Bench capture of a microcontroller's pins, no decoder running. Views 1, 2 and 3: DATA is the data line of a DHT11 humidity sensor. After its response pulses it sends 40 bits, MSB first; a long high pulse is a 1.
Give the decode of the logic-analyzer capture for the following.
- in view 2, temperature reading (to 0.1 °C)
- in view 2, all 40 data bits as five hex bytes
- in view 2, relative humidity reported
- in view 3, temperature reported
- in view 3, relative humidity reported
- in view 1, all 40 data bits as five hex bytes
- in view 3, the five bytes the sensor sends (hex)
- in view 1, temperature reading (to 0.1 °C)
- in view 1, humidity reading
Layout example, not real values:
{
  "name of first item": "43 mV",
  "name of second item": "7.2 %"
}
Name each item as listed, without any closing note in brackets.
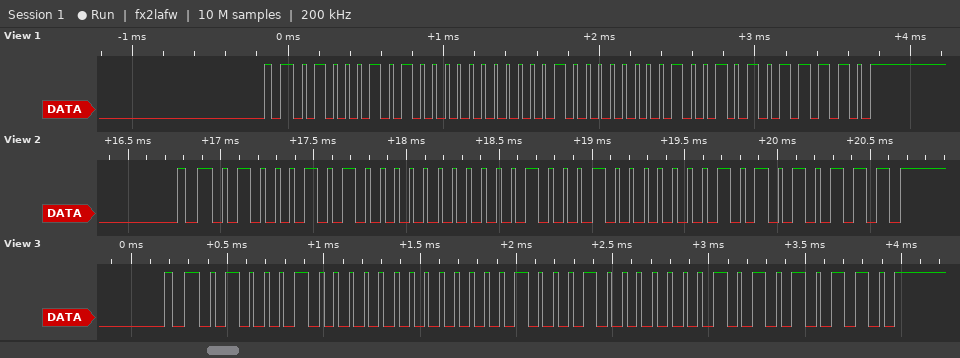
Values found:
{
  "in view 2, temperature reading": "17.1 °C",
  "in view 2, all 40 data bits as five hex bytes": "45 00 11 01 57",
  "in view 2, relative humidity reported": "69 %",
  "in view 3, temperature reported": "17.1 °C",
  "in view 3, relative humidity reported": "68 %",
  "in view 1, all 40 data bits as five hex bytes": "45 00 10 09 5E",
  "in view 3, the five bytes the sensor sends": "44 00 11 01 56",
  "in view 1, temperature reading": "16.9 °C",
  "in view 1, humidity reading": "69 %"
}
